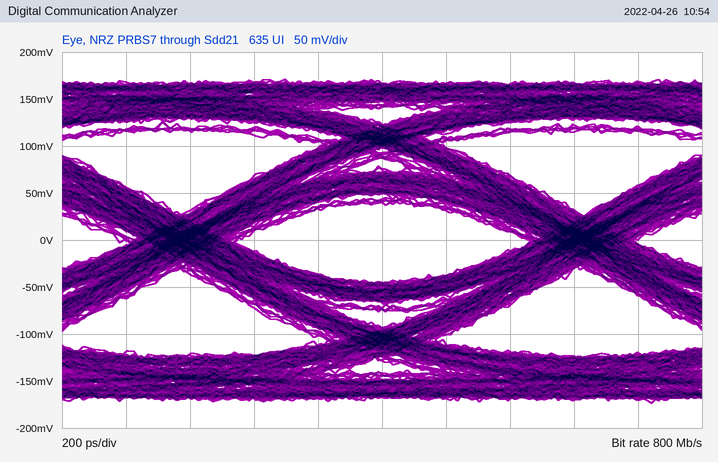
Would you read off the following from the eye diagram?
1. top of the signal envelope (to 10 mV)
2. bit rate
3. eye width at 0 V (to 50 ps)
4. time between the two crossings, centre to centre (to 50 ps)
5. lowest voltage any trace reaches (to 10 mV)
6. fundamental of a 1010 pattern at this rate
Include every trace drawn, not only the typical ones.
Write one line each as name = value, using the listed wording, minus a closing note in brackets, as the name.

top of the signal envelope = 170 mV
bit rate = 800 Mb/s
eye width at 0 V = 900 ps
time between the two crossings, centre to centre = 1.25 ns
lowest voltage any trace reaches = -170 mV
fundamental of a 1010 pattern at this rate = 400 MHz
